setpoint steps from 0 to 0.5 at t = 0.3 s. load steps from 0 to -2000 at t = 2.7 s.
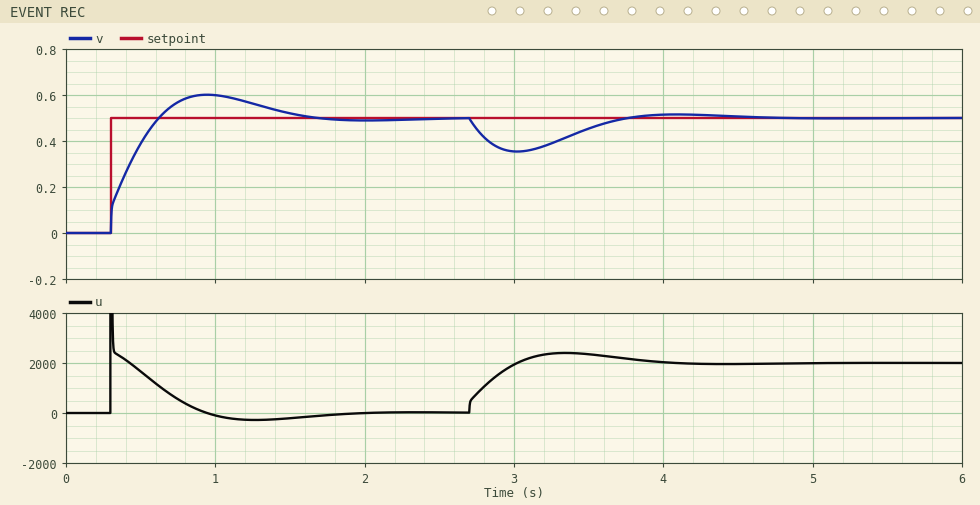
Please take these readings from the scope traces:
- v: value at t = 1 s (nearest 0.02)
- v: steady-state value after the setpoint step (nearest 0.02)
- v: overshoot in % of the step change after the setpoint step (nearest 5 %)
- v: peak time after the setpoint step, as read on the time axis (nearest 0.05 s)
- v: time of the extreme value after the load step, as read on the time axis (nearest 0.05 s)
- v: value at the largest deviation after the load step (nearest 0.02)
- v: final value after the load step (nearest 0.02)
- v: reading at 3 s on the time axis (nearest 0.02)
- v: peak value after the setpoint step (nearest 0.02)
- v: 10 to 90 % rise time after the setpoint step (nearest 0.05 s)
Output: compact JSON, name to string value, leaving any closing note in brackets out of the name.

{"v: value at t = 1 s": "0.60", "v: steady-state value after the setpoint step": "0.50", "v: overshoot in % of the step change after the setpoint step": "20 %", "v: peak time after the setpoint step, as read on the time axis": "0.95 s", "v: time of the extreme value after the load step, as read on the time axis": "3.00 s", "v: value at the largest deviation after the load step": "0.36", "v: final value after the load step": "0.50", "v: reading at 3 s on the time axis": "0.36", "v: peak value after the setpoint step": "0.60", "v: 10 to 90 % rise time after the setpoint step": "0.25 s"}
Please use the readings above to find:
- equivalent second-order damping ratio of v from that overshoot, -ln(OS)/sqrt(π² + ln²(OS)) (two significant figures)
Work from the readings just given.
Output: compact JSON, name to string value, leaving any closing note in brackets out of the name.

{"equivalent second-order damping ratio of v from that overshoot, -ln(OS)/sqrt(π² + ln²(OS))": "0.46"}
